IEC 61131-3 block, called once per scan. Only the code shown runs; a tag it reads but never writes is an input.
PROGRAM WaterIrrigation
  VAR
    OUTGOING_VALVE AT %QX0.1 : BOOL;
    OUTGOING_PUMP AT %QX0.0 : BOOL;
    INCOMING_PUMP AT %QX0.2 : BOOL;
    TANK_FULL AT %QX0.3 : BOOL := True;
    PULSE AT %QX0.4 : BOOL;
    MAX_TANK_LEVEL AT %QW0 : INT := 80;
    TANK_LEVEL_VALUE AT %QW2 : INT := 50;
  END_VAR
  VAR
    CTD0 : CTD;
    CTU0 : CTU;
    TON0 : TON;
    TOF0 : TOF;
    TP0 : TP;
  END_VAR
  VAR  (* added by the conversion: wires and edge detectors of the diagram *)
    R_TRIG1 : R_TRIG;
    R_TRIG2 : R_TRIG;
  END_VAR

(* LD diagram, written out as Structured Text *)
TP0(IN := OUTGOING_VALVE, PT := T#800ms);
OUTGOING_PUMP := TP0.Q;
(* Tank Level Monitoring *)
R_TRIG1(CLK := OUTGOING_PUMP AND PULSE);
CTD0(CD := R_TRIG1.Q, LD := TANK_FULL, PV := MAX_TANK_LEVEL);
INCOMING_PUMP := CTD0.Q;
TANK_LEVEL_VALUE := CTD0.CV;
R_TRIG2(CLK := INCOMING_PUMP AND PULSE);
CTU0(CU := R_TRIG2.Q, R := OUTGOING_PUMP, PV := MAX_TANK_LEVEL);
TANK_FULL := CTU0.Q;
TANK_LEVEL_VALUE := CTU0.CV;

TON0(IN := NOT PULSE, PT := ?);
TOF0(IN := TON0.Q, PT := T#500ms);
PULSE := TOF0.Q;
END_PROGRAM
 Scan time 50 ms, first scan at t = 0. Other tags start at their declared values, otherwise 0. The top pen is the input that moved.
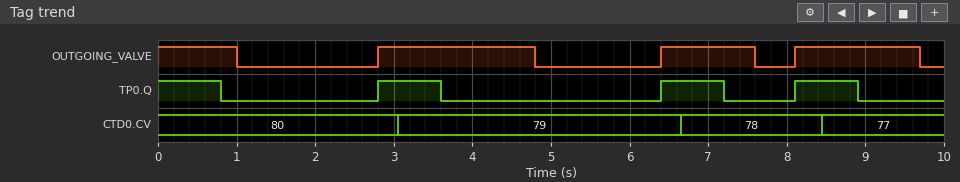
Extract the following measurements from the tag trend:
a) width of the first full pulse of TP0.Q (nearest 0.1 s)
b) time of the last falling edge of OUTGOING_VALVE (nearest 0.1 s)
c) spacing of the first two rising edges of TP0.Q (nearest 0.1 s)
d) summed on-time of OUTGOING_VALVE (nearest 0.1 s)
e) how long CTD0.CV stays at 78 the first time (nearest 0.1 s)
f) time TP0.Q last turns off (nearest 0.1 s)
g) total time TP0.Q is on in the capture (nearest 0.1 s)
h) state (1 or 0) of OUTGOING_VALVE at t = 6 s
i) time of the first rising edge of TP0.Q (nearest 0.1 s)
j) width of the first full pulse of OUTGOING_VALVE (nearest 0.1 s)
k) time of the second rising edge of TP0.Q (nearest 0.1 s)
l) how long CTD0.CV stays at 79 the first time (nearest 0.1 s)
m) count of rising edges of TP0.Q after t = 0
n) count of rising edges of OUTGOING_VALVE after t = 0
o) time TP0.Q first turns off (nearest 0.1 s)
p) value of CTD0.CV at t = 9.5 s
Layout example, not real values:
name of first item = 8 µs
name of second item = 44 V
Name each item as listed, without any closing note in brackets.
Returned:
width of the first full pulse of TP0.Q = 0.8 s
time of the last falling edge of OUTGOING_VALVE = 9.7 s
spacing of the first two rising edges of TP0.Q = 3.6 s
summed on-time of OUTGOING_VALVE = 5.8 s
how long CTD0.CV stays at 78 the first time = 1.8 s
time TP0.Q last turns off = 8.9 s
total time TP0.Q is on in the capture = 3.2 s
state (1 or 0) of OUTGOING_VALVE at t = 6 s = 0
time of the first rising edge of TP0.Q = 2.8 s
width of the first full pulse of OUTGOING_VALVE = 2.0 s
time of the second rising edge of TP0.Q = 6.4 s
how long CTD0.CV stays at 79 the first time = 3.6 s
count of rising edges of TP0.Q after t = 0 = 3
count of rising edges of OUTGOING_VALVE after t = 0 = 3
time TP0.Q first turns off = 0.8 s
value of CTD0.CV at t = 9.5 s = 77
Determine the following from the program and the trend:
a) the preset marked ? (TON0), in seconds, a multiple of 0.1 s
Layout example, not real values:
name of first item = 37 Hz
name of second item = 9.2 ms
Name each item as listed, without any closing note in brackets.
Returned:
the preset marked ? (TON0), in seconds, a multiple of 0.1 s = 1.2 s
